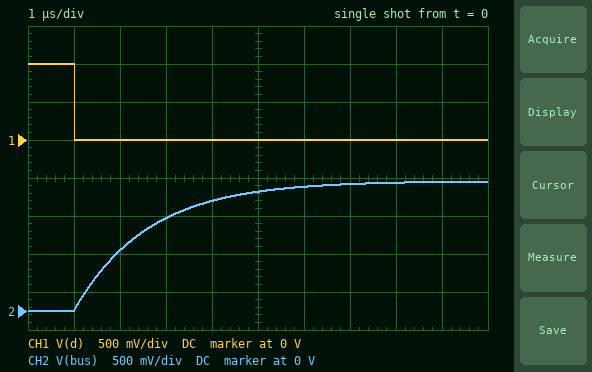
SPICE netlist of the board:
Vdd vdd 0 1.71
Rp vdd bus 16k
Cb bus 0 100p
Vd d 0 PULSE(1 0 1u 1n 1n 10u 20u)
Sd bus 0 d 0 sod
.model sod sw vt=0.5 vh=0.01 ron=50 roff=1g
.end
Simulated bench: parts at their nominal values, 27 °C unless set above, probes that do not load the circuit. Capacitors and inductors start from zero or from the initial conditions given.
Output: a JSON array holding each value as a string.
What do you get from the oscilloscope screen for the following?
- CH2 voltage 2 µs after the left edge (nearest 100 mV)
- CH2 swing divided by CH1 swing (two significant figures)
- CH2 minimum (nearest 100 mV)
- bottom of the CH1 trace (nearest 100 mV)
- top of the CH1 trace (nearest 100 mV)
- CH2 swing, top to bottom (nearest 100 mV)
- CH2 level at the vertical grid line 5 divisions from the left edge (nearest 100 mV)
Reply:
["800 mV", "1.7", "0 V", "0 V", "1.0 V", "1.7 V", "1.6 V"]
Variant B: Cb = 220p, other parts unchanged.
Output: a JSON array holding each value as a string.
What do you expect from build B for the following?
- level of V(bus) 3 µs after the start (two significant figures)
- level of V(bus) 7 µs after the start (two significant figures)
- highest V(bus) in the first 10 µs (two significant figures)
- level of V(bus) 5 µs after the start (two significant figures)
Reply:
["740 mV", "1.4 V", "1.6 V", "1.2 V"]
